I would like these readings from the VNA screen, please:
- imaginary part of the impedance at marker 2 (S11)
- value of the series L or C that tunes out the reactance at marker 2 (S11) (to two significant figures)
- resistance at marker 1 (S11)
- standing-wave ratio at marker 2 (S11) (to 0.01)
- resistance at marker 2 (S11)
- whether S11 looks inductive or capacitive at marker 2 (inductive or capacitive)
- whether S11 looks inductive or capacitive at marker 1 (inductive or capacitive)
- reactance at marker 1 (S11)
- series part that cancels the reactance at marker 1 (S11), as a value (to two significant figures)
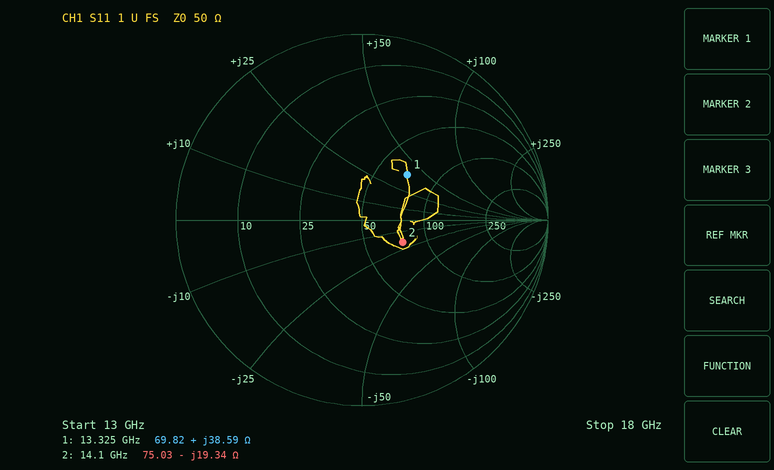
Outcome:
-19.34 Ω
220 pH
69.82 Ω
1.67
75.03 Ω
capacitive
inductive
+38.59 Ω
310 fF
